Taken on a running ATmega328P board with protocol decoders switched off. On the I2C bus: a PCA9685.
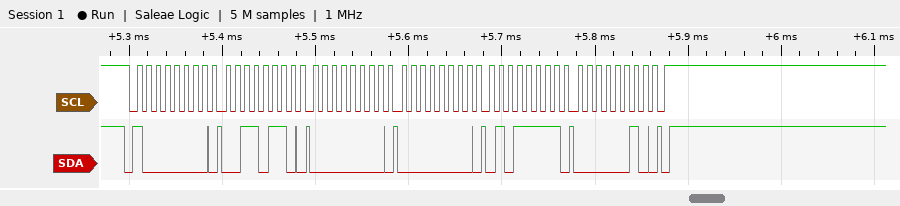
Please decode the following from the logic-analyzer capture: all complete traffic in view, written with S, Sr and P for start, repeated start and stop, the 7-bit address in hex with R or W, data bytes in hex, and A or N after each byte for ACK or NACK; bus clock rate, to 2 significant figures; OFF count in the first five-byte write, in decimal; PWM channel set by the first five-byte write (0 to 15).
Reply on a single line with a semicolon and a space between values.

S 40W A 36 A 00 A 00 A 5F A 02 A P; 100 kHz; 607; 12
